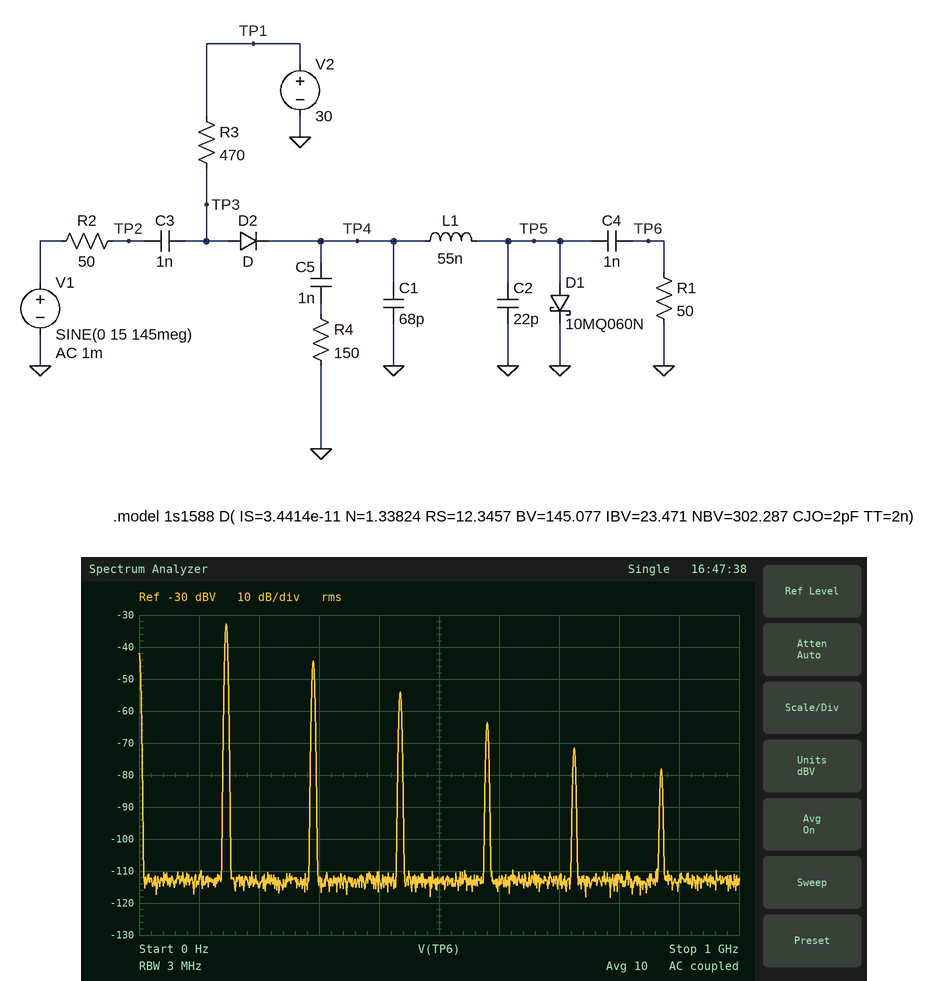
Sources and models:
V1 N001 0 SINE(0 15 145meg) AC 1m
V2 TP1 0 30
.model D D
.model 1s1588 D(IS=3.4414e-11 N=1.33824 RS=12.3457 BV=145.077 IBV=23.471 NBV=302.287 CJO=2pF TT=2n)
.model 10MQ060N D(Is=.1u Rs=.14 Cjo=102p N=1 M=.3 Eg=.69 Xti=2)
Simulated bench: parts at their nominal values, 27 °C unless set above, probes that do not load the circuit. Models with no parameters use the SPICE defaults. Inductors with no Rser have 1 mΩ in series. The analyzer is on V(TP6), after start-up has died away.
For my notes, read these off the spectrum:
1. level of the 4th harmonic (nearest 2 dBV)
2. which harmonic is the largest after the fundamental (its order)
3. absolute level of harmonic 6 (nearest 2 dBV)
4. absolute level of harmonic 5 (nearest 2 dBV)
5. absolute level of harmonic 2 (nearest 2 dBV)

-64 dBV
2
-78 dBV
-72 dBV
-44 dBV
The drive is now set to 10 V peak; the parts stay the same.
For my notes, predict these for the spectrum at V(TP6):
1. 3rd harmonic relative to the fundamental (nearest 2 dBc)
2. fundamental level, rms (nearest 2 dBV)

-24 dBc
-34 dBV
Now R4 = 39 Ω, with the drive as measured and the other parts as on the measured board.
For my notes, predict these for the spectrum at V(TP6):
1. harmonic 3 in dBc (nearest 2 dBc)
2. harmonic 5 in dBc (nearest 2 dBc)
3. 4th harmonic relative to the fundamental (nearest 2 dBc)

-24 dBc
-46 dBc
-36 dBc
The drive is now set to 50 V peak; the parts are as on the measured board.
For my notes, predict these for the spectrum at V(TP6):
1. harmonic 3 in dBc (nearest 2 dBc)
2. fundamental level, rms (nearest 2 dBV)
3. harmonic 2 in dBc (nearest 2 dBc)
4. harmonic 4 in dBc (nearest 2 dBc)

-16 dBc
-30 dBV
-10 dBc
-22 dBc
